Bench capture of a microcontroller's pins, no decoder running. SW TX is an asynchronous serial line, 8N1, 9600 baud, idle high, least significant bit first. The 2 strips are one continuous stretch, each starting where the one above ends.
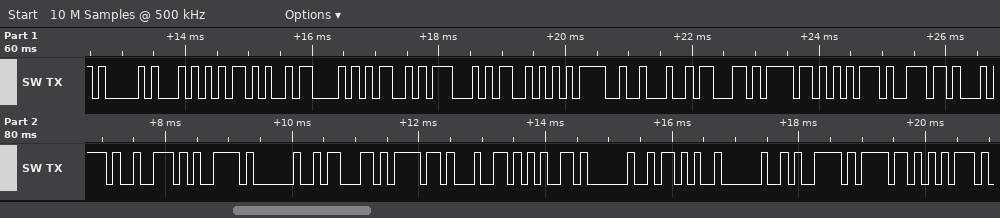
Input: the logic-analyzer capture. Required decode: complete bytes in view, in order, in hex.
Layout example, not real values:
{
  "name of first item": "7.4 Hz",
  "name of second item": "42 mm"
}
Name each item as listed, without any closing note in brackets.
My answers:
{
  "complete bytes in view, in order, in hex": "41 54 2B 43 4D 47 53 3D 22 63 6F 75 6E 74 72 79 20 63 6F 64 65 20 2B 20 79 6F 75"
}
